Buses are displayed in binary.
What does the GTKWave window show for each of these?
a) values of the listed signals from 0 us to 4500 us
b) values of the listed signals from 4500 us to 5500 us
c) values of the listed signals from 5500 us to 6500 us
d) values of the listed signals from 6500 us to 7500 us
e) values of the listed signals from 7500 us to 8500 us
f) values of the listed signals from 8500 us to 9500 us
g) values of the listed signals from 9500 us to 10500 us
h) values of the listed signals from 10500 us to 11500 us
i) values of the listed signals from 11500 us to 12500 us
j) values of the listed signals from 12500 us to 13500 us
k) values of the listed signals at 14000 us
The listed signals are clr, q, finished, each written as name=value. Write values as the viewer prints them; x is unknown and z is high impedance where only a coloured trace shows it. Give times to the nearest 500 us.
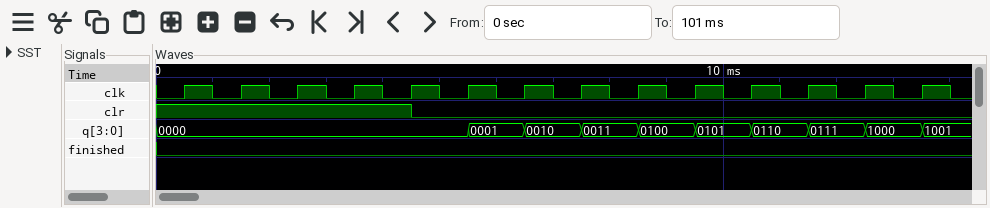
clr=1, q=0000, finished=0
clr=0, q=0000, finished=0
clr=0, q=0001, finished=0
clr=0, q=0010, finished=0
clr=0, q=0011, finished=0
clr=0, q=0100, finished=0
clr=0, q=0101, finished=0
clr=0, q=0110, finished=0
clr=0, q=0111, finished=0
clr=0, q=1000, finished=0
clr=0, q=1001, finished=0
